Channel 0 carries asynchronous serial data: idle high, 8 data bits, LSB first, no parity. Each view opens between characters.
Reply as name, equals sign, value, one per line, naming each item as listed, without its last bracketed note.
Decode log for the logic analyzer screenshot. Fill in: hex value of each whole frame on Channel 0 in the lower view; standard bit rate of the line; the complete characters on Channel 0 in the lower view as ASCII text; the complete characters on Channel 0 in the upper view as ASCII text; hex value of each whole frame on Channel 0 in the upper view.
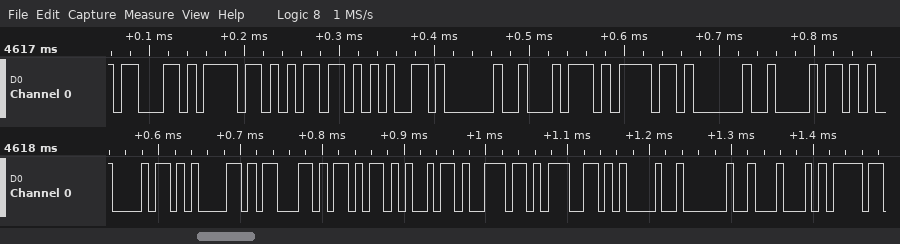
hex value of each whole frame on Channel 0 in the lower view = 68, 61, 63, 6B, 69, 6E, 67, 21, 20, 44
standard bit rate of the line = 115200 baud
the complete characters on Channel 0 in the lower view as ASCII text = "hacking! D"
the complete characters on Channel 0 in the upper view as ASCII text = "come to h"
hex value of each whole frame on Channel 0 in the upper view = 63, 6F, 6D, 65, 20, 74, 6F, 20, 68
